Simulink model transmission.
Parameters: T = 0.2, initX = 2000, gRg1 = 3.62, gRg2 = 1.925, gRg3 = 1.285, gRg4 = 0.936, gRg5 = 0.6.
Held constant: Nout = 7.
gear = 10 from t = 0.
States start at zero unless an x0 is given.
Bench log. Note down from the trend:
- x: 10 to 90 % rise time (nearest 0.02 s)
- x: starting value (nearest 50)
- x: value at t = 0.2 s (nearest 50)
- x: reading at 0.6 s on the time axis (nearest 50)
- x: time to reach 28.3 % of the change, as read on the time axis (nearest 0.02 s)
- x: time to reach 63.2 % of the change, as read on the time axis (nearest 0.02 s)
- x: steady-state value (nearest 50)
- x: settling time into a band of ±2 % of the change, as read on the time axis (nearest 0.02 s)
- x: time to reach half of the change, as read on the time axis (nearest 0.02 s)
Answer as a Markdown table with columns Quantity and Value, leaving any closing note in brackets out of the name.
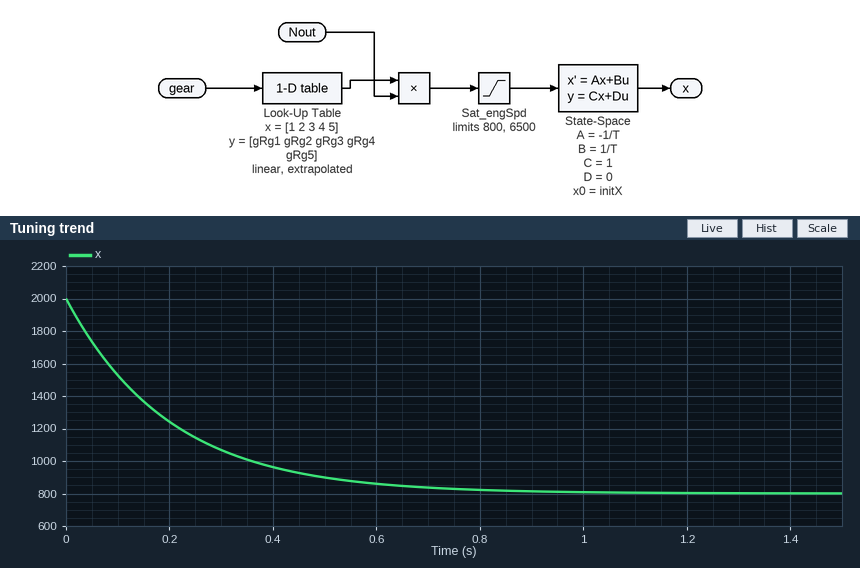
| Quantity | Value |
|---|---|
| x: 10 to 90 % rise time | 0.44 s |
| x: starting value | 2000 |
| x: value at t = 0.2 s | 1250 |
| x: reading at 0.6 s on the time axis | 850 |
| x: time to reach 28.3 % of the change, as read on the time axis | 0.06 s |
| x: time to reach 63.2 % of the change, as read on the time axis | 0.20 s |
| x: steady-state value | 800 |
| x: settling time into a band of ±2 % of the change, as read on the time axis | 0.78 s |
| x: time to reach half of the change, as read on the time axis | 0.14 s |
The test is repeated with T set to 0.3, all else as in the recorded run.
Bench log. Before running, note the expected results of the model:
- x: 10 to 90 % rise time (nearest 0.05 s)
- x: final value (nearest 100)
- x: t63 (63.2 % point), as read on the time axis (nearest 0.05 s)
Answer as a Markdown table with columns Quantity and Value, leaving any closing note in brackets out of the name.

| Quantity | Value |
|---|---|
| x: 10 to 90 % rise time | 0.65 s |
| x: final value | 800 |
| x: t63 (63.2 % point), as read on the time axis | 0.30 s |
